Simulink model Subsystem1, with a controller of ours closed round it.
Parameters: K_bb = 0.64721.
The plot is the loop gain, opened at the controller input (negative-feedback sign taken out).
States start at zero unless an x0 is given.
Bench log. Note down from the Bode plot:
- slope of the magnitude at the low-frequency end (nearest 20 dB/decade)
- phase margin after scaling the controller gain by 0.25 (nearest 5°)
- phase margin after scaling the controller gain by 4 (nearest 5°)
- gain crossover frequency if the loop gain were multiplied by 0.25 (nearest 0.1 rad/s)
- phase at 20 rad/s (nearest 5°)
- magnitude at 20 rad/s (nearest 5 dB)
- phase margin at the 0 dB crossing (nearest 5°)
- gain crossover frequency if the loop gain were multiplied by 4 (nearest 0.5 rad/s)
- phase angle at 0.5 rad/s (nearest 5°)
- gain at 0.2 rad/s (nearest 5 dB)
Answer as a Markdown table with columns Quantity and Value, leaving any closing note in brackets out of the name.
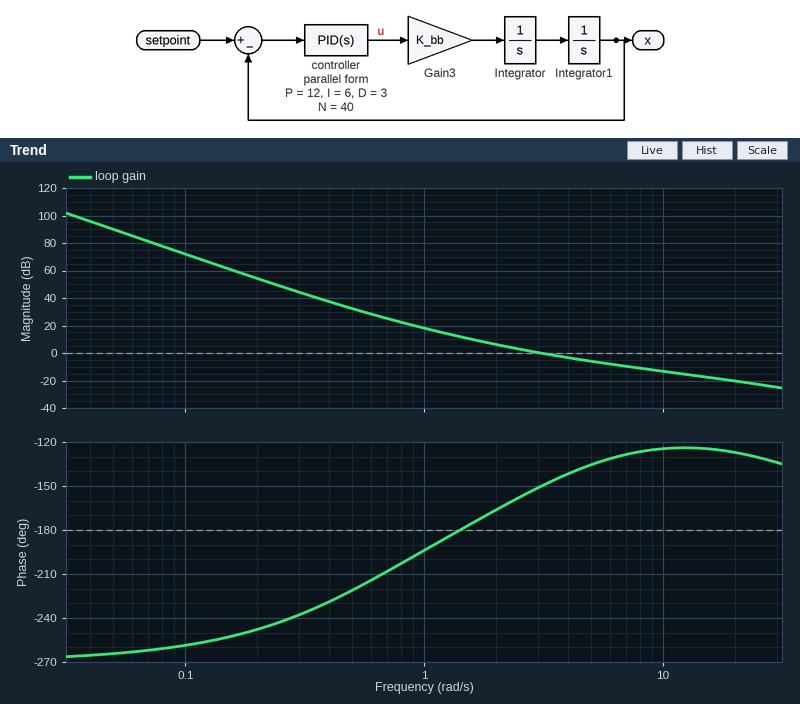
| Quantity | Value |
|---|---|
| slope of the magnitude at the low-frequency end | -60 dB/decade |
| phase margin after scaling the controller gain by 0.25 | 0° |
| phase margin after scaling the controller gain by 4 | 55° |
| gain crossover frequency if the loop gain were multiplied by 0.25 | 1.4 rad/s |
| phase at 20 rad/s | -125° |
| magnitude at 20 rad/s | -20 dB |
| phase margin at the 0 dB crossing | 30° |
| gain crossover frequency if the loop gain were multiplied by 4 | 9.0 rad/s |
| phase angle at 0.5 rad/s | -220° |
| gain at 0.2 rad/s | 55 dB |
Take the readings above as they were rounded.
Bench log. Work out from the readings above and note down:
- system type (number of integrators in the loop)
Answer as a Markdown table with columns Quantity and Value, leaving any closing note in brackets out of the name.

| Quantity | Value |
|---|---|
| system type | 3 |
